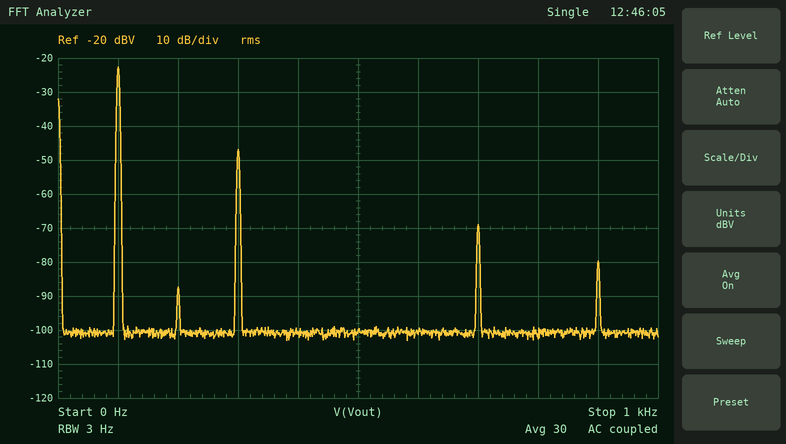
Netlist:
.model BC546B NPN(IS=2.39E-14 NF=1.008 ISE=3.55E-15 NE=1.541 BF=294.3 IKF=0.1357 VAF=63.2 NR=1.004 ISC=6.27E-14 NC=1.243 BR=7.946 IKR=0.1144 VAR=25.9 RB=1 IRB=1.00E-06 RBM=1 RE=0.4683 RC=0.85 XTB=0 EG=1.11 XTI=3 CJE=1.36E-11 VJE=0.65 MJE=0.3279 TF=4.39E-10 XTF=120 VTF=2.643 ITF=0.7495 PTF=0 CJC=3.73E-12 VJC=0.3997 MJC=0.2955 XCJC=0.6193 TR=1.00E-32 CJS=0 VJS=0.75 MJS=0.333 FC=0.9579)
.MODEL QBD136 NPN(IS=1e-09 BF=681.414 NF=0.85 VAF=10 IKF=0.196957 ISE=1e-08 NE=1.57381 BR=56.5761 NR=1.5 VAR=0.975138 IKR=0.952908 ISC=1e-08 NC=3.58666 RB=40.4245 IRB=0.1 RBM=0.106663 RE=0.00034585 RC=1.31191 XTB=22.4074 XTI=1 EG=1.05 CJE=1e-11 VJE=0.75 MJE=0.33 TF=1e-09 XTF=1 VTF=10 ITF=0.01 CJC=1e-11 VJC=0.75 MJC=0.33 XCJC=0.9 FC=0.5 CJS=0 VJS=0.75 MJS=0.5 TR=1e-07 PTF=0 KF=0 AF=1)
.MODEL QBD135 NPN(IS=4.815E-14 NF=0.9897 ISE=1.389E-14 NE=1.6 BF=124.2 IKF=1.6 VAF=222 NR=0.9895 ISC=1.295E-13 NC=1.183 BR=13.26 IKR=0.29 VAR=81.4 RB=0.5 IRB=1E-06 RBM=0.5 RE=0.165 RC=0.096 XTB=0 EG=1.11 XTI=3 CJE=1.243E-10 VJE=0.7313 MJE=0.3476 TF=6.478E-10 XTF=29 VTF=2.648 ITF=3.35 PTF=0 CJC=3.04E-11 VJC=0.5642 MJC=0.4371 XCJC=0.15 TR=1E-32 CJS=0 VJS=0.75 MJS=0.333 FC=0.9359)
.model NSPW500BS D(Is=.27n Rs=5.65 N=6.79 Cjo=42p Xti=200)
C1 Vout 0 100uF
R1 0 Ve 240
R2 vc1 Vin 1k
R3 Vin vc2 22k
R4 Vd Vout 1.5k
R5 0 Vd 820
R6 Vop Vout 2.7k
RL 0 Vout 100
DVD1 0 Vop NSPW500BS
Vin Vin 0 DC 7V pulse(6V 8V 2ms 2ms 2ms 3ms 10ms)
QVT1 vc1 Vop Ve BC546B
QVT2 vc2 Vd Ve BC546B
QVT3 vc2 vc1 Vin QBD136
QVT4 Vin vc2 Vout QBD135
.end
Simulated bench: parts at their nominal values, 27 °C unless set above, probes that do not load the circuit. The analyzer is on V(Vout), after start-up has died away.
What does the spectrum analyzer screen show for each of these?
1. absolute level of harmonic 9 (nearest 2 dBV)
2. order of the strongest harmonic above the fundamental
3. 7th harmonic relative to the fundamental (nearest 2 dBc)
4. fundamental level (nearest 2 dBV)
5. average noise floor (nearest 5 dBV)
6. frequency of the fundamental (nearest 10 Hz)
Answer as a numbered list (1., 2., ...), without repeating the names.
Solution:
1. -80 dBV
2. 3
3. -46 dBc
4. -22 dBV
5. -100 dBV
6. 100 Hz
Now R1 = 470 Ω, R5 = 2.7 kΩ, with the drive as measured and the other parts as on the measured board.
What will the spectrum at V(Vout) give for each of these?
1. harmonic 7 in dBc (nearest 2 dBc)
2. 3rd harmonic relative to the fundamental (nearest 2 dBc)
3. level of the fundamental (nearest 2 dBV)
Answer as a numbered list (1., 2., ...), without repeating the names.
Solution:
1. -42 dBc
2. -14 dBc
3. -16 dBV
